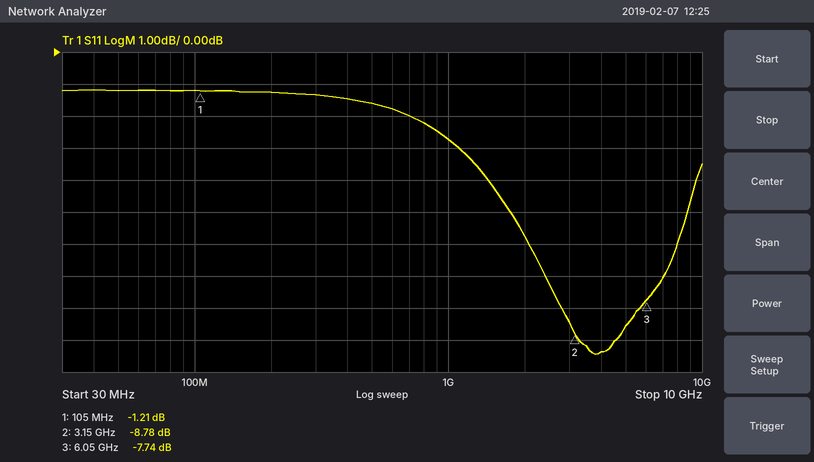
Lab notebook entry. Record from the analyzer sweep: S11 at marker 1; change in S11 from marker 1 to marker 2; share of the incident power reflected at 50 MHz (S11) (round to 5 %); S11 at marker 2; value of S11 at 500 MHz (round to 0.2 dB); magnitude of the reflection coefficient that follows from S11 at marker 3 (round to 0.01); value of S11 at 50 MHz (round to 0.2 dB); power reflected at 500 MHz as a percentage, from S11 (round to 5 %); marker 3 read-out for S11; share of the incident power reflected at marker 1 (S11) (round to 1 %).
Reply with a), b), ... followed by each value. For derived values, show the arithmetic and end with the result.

a) -1.21 dB
b) -8.78 − (-1.21) = -7.57 dB
c) 10^(-1.2/10) ≈ 75.9 %, so 75 % to the nearest 5 %
d) -8.78 dB
e) -1.6 dB
f) 10^(-7.74/20) ≈ 0.41
g) -1.2 dB
h) 10^(-1.6/10) ≈ 69.2 %, so 70 % to the nearest 5 %
i) -7.74 dB
j) 10^(-1.21/10) ≈ 76 %
